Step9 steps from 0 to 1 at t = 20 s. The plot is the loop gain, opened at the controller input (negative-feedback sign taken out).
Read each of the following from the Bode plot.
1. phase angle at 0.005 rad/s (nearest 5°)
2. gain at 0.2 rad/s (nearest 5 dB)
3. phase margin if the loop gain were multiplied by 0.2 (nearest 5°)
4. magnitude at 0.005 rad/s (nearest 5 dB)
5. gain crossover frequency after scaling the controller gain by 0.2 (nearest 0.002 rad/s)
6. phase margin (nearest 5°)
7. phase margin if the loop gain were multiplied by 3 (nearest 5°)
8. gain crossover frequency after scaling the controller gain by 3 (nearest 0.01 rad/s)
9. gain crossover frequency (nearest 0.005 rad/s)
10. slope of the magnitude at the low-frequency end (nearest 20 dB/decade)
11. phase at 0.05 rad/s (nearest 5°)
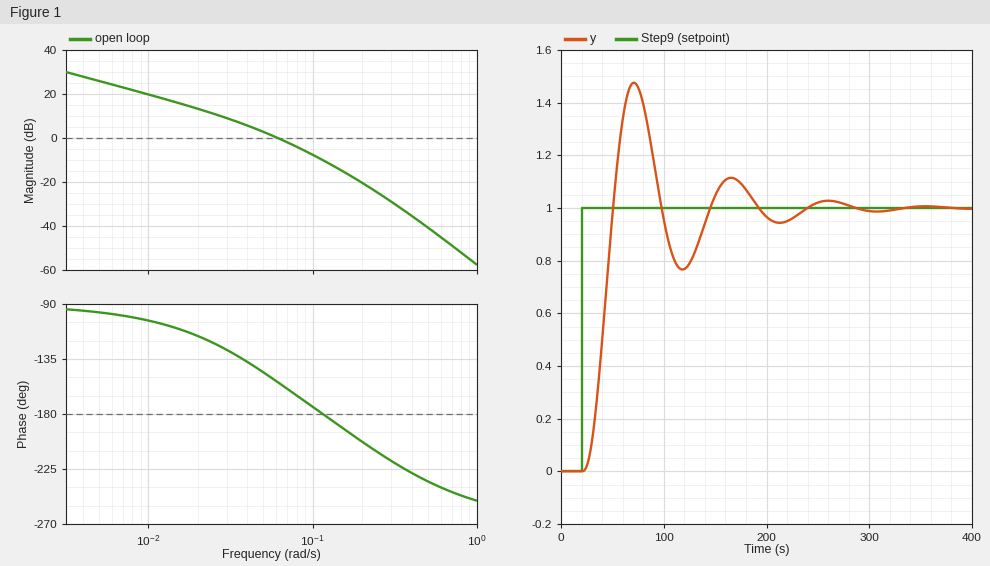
-95°
-20 dB
65°
25 dB
0.018 rad/s
25°
0°
0.11 rad/s
0.060 rad/s
-20 dB/decade
-145°
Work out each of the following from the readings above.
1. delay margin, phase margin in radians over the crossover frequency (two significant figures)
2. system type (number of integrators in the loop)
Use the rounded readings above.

7.3 s
1
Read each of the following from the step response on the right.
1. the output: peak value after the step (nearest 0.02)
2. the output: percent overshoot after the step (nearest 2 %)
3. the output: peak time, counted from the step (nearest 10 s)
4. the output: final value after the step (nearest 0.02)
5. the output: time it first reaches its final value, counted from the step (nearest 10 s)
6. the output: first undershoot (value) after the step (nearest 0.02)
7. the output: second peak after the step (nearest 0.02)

1.48
48 %
50 s
1.00
30 s
0.76
1.12
